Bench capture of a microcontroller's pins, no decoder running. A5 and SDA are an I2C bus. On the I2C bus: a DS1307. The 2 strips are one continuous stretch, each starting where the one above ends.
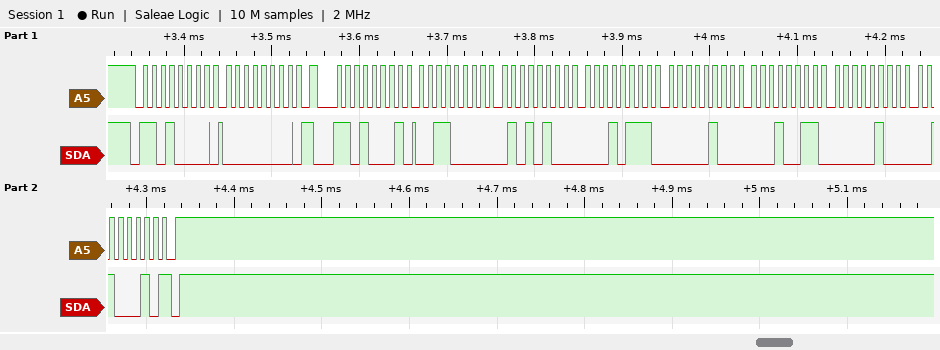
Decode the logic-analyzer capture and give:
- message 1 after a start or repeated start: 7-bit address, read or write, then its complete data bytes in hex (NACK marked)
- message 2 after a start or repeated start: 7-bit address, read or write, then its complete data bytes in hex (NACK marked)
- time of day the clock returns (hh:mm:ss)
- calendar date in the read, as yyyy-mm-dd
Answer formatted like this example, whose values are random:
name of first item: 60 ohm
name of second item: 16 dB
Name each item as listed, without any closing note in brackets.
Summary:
message 1 after a start or repeated start: 7-bit address, read or write, then its complete data bytes in hex: 0x68 write: 00
message 2 after a start or repeated start: 7-bit address, read or write, then its complete data bytes in hex: 0x68 read: 30 54 17 04 13 04 22 NACK
time of day the clock returns: 17:54:30
calendar date in the read, as yyyy-mm-dd: 2022-04-13
